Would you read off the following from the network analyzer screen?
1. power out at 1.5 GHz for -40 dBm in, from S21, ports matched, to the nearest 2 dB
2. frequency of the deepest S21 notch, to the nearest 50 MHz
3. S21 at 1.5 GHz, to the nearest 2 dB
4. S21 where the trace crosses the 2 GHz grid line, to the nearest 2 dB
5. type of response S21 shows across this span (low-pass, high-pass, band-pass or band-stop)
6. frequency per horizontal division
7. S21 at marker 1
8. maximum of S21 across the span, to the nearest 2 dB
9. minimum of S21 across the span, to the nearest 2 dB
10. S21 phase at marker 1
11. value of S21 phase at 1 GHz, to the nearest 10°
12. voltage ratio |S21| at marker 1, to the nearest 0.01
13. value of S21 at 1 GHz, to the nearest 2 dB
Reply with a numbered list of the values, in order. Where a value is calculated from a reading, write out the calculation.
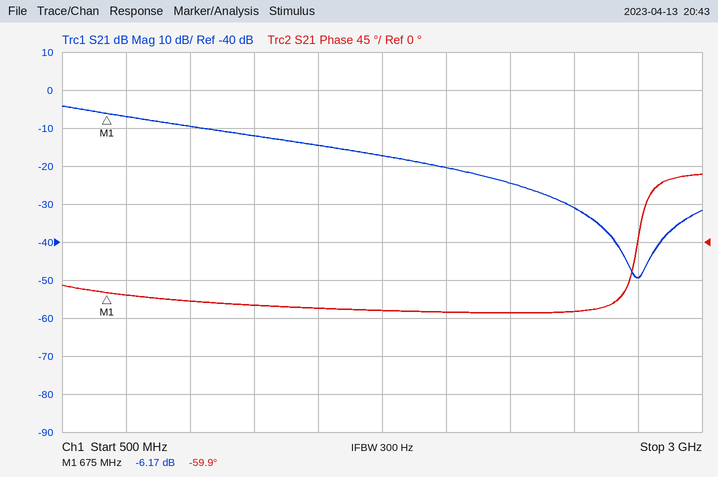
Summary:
1. -40 dBm + (-14 dB) = -54 dBm
2. 2.75 GHz
3. -14 dB
4. -20 dB
5. low-pass
6. 250 MHz
7. -6.17 dB
8. -4 dB
9. -50 dB
10. -59.9°
11. -70°
12. 10^(-6.17/20) ≈ 0.49
13. -10 dB
